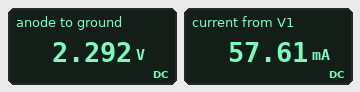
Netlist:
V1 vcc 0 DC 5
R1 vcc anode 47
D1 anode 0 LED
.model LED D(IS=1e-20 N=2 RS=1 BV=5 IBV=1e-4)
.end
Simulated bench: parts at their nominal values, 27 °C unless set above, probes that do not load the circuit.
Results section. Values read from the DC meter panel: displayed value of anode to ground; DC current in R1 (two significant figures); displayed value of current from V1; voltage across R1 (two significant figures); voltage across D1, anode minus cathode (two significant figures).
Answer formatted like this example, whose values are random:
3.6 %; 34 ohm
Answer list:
2.292 V; 58 mA; 57.61 mA; 2.7 V; 2.3 V
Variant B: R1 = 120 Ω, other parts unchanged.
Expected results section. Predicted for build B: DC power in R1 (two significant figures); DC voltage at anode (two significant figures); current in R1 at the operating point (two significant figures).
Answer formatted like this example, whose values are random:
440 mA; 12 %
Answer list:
65 mW; 2.2 V; 23 mA
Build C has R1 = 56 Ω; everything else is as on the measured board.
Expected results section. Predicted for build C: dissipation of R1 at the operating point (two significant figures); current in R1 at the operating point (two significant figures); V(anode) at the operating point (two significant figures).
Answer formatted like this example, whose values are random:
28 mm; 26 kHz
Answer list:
130 mW; 49 mA; 2.3 V
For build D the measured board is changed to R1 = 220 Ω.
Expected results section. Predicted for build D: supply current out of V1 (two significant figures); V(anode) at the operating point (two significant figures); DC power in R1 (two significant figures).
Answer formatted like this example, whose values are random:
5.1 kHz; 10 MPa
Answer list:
13 mA; 2.2 V; 36 mW
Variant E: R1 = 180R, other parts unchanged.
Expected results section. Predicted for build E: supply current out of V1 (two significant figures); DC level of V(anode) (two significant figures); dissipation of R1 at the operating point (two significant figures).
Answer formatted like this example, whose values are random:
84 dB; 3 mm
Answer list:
16 mA; 2.2 V; 44 mW
